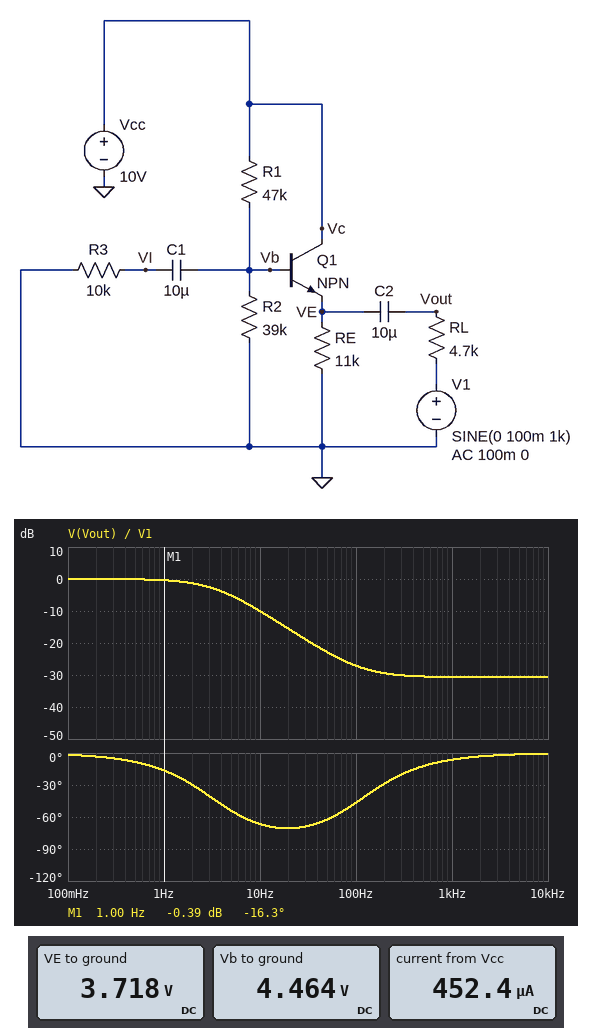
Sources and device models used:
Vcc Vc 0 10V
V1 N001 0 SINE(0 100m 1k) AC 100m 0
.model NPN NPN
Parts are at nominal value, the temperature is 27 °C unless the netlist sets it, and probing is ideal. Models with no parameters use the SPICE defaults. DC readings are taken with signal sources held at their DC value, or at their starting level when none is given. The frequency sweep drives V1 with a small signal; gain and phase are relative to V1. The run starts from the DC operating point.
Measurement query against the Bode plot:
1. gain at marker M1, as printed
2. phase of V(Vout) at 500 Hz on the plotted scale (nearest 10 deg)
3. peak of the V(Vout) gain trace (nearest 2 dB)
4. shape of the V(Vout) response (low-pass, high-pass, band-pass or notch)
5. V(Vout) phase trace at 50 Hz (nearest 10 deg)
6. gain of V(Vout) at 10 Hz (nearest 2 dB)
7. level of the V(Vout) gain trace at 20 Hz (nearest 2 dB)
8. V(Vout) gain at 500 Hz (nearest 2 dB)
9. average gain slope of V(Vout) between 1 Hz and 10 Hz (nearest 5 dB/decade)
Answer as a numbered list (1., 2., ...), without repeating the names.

1. -0.39 dB
2. -10 deg
3. 0 dB
4. low-pass
5. -60 deg
6. -10 dB
7. -16 dB
8. -30 dB
9. -10 dB/decade
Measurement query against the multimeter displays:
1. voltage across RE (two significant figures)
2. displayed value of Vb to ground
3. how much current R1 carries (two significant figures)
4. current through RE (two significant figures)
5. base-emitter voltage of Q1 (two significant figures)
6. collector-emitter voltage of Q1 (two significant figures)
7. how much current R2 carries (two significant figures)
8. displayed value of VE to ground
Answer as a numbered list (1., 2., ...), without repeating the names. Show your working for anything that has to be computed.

1. 3.718 V = 3.7 V
2. 4.464 V
3. (10 V - 4.464 V) / 47 kΩ = 120 µA
4. (3.718 V) / 11 kΩ = 340 µA
5. 4.464 V - 3.718 V = 750 mV
6. 10 V - 3.718 V = 6.3 V
7. (4.464 V) / 39 kΩ = 110 µA
8. 3.718 V
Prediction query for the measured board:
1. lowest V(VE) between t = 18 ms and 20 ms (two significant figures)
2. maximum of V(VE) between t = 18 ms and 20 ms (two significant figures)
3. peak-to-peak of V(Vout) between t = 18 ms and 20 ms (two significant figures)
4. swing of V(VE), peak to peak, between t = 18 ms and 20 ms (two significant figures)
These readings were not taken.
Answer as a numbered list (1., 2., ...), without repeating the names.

1. 3.7 V
2. 3.7 V
3. 5.9 mV
4. 5.9 mV
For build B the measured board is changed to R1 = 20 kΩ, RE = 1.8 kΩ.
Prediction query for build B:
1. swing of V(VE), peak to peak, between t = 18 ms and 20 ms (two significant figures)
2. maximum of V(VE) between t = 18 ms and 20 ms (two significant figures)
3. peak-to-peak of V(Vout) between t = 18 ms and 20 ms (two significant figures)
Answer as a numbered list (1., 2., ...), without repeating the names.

1. 2.6 mV
2. 5.4 V
3. 2.7 mV
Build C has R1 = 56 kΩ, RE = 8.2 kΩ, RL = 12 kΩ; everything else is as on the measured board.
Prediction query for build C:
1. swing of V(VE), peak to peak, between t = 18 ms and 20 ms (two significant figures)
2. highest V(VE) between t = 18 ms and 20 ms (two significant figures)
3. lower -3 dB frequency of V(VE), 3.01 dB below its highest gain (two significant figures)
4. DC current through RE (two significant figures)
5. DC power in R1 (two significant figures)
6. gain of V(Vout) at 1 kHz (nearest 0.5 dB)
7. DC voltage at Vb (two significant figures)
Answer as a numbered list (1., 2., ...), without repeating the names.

1. 2.2 mV
2. 3.3 V
3. 730 mHz
4. 400 µA
5. 640 µW
6. -39.0 dB
7. 4.0 V
